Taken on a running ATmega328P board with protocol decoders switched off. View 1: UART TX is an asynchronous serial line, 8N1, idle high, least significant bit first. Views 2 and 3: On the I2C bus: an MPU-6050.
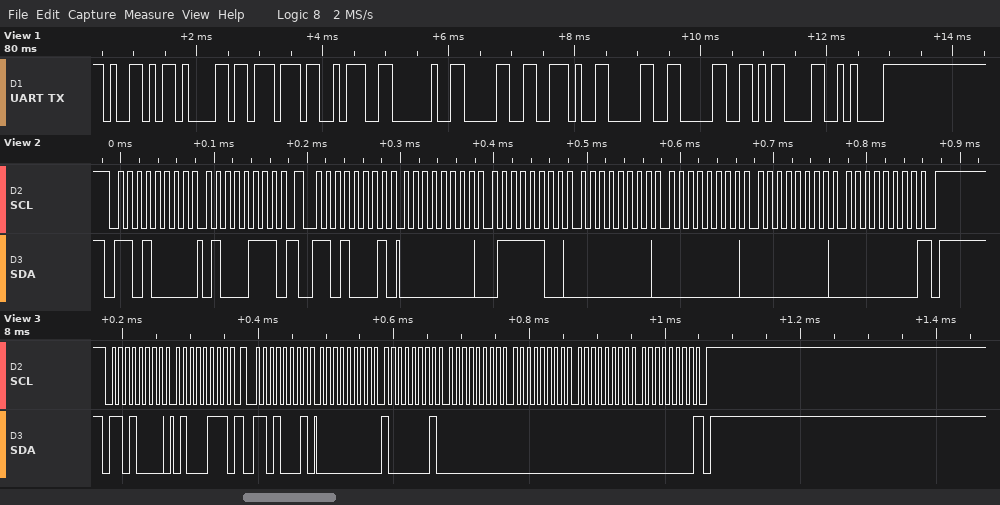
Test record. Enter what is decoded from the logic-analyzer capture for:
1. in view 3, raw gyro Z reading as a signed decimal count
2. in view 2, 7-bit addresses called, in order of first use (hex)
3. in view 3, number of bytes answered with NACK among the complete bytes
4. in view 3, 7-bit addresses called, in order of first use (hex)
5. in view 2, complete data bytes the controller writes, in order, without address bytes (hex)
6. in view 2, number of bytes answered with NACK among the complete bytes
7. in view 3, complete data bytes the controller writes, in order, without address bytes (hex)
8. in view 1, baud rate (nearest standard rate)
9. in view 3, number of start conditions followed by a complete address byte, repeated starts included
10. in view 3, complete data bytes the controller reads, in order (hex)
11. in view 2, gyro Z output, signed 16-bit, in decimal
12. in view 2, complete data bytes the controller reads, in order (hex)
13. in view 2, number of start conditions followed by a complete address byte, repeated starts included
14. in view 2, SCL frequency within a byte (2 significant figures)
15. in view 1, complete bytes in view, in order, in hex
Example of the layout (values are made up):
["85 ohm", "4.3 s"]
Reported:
["129", "0x68", "1", "0x68", "47", "1", "47", "9600 baud", "2", "00 81 00 00 00 00", "124", "00 7C 00 00 00 00", "2", "100 kHz", "59 61 77 3A 20 30 2E 30 30 0D 0A"]
